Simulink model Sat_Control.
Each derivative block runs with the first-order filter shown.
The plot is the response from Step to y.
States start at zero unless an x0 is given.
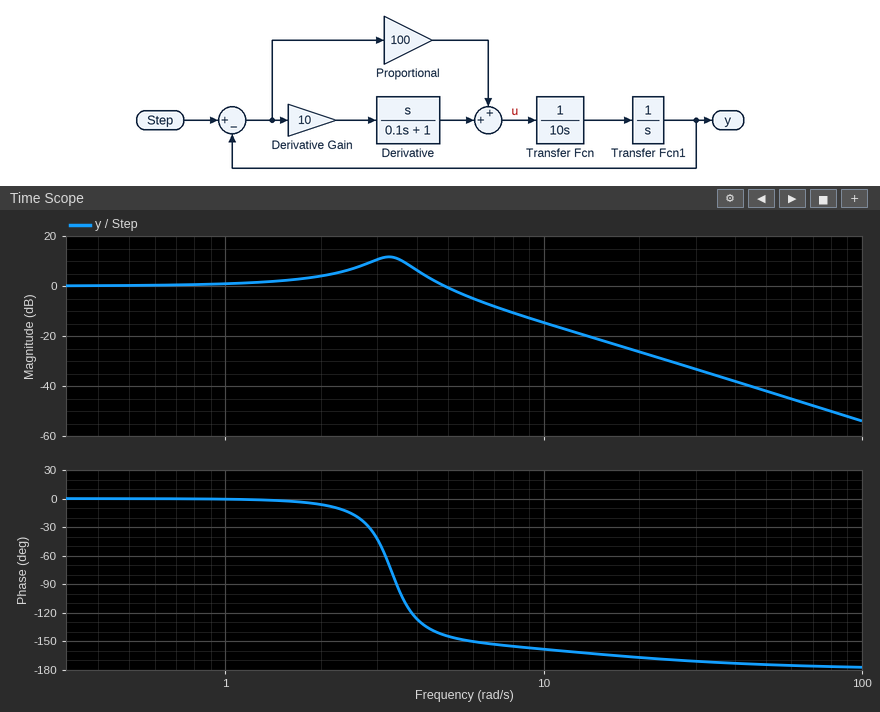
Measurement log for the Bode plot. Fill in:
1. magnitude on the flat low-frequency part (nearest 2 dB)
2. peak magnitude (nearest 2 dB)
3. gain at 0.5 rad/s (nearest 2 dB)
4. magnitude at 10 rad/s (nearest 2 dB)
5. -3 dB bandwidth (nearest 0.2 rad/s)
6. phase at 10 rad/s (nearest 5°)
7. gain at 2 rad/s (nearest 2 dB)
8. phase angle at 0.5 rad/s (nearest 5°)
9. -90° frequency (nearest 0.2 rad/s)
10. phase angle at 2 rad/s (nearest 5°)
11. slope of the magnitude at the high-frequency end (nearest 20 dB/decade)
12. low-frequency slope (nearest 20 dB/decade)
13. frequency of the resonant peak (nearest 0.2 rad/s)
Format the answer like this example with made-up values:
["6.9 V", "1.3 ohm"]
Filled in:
["0 dB", "12 dB", "0 dB", "-14 dB", "5.4 rad/s", "-160°", "4 dB", "0°", "3.4 rad/s", "-5°", "-40 dB/decade", "0 dB/decade", "3.2 rad/s"]
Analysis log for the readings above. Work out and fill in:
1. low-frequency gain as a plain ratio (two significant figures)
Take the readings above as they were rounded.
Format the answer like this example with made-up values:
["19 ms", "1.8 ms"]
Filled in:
["1.0"]
